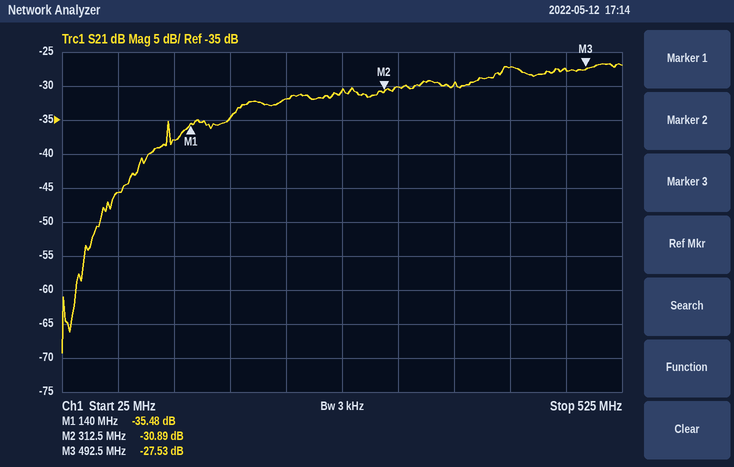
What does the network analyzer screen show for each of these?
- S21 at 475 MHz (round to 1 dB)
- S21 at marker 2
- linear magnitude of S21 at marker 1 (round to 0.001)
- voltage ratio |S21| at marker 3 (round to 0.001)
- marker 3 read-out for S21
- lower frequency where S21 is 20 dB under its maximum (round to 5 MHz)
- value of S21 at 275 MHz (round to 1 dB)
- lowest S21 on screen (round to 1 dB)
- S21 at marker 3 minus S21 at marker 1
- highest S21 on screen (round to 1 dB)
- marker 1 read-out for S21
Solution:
-28 dB
-30.89 dB
0.017
0.042
-27.53 dB
70 MHz
-31 dB
-69 dB
7.95 dB
-27 dB
-35.48 dB
